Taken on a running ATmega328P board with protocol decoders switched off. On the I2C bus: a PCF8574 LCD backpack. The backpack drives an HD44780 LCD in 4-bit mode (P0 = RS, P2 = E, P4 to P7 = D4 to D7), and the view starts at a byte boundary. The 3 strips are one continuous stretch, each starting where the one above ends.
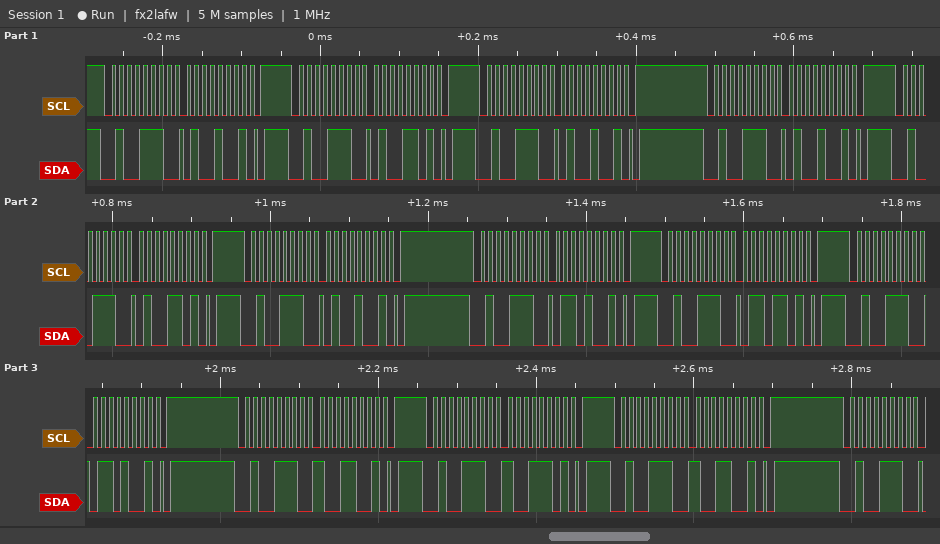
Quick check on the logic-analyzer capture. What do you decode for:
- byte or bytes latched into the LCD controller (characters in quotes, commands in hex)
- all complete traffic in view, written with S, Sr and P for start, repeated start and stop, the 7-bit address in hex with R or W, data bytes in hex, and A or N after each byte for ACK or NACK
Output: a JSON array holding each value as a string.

["'D' 'i'", "S 27W A 49 A P S 27W A 4D A P S 27W A 49 A P S 27W A 49 A P S 27W A 4D A P S 27W A 49 A P S 27W A 69 A P S 27W A 6D A P S 27W A 69 A P S 27W A 99 A P S 27W A 9D A P S 27W A 99 A P S 27W A"]
